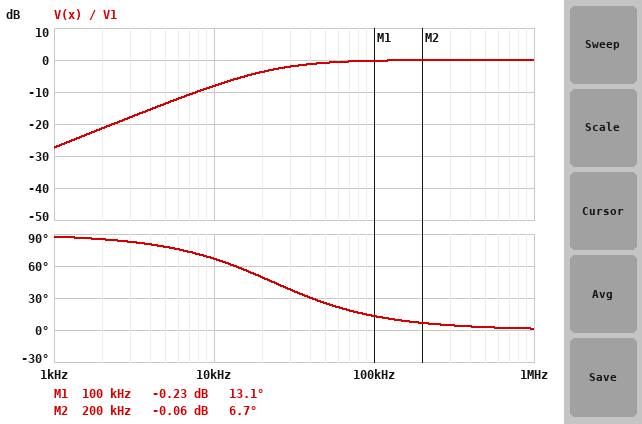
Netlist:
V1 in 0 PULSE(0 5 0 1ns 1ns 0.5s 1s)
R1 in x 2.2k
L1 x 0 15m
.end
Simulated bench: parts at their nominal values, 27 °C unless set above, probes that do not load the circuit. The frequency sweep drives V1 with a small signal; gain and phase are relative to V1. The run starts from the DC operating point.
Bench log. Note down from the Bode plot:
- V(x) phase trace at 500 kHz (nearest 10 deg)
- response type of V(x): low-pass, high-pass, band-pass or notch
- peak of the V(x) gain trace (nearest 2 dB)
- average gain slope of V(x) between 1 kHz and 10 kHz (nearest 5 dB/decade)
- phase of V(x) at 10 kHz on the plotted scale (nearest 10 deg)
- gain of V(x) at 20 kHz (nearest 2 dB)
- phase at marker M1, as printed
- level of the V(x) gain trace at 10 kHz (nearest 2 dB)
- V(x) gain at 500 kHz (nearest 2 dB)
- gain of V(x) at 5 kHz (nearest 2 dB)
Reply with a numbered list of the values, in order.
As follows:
1. 0 deg
2. high-pass
3. 0 dB
4. 20 dB/decade
5. 70 deg
6. -4 dB
7. 13.1 deg
8. -8 dB
9. 0 dB
10. -14 dB
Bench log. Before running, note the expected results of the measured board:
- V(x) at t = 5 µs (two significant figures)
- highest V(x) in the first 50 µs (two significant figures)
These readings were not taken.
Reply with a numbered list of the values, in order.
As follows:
1. 2.4 V
2. 5.0 V
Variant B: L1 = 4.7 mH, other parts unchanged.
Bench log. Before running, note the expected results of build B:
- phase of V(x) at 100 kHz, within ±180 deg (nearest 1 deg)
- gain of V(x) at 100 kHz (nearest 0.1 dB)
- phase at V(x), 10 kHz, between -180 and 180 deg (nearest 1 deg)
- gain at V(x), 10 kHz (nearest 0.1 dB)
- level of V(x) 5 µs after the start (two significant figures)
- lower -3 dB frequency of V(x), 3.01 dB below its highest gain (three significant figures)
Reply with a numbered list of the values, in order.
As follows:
1. 37 deg
2. -1.9 dB
3. 82 deg
4. -17.5 dB
5. 480 mV
6. 74.5 kHz
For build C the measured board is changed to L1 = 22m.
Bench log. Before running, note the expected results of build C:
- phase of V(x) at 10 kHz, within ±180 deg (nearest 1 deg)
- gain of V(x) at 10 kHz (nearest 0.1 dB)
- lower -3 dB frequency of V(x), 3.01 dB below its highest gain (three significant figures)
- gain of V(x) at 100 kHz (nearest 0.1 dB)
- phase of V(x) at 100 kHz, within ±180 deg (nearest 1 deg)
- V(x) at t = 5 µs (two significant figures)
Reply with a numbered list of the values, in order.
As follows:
1. 58 deg
2. -5.5 dB
3. 15.9 kHz
4. -0.1 dB
5. 9 deg
6. 3.0 V
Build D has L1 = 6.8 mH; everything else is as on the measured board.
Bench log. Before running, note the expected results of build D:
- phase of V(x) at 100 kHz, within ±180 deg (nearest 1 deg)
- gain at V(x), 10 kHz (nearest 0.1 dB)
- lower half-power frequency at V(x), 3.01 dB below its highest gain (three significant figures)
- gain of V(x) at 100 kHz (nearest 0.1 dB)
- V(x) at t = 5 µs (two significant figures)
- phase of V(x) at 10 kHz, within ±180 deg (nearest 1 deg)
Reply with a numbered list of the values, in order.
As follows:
1. 27 deg
2. -14.4 dB
3. 51.5 kHz
4. -1.0 dB
5. 990 mV
6. 79 deg
